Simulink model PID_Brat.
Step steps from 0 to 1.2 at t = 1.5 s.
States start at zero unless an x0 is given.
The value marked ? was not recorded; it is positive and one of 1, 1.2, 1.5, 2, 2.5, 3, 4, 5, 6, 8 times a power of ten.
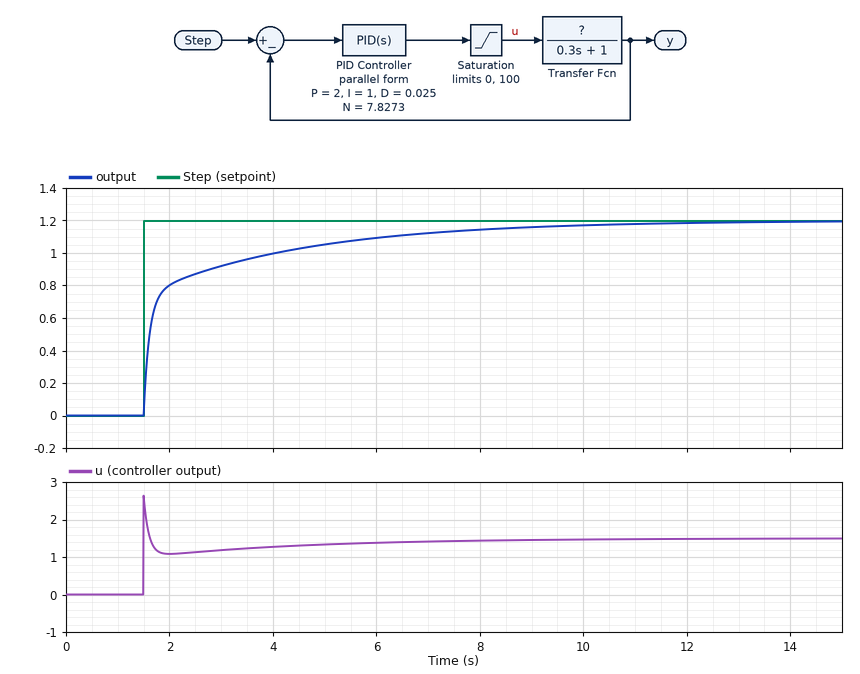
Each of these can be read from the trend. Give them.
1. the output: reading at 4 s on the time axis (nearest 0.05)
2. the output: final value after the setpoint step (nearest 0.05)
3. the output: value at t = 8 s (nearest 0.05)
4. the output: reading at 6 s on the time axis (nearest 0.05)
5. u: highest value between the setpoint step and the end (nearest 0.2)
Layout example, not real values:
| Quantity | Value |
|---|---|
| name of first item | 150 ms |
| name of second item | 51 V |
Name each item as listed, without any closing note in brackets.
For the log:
| Quantity | Value |
|---|---|
| the output: reading at 4 s on the time axis | 1.00 |
| the output: final value after the setpoint step | 1.20 |
| the output: value at t = 8 s | 1.15 |
| the output: reading at 6 s on the time axis | 1.10 |
| u: highest value between the setpoint step and the end | 2.6 |
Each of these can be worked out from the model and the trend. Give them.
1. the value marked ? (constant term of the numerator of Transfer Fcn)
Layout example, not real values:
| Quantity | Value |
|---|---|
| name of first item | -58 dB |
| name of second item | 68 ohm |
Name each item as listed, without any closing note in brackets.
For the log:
| Quantity | Value |
|---|---|
| the value marked ? | 0.8 |
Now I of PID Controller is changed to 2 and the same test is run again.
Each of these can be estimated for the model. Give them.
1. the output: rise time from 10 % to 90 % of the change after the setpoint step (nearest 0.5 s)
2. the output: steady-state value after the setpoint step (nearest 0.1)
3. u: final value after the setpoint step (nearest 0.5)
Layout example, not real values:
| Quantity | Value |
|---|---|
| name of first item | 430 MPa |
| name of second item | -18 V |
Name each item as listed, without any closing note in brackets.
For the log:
| Quantity | Value |
|---|---|
| the output: rise time from 10 % to 90 % of the change after the setpoint step | 2.0 s |
| the output: steady-state value after the setpoint step | 1.2 |
| u: final value after the setpoint step | 1.5 |
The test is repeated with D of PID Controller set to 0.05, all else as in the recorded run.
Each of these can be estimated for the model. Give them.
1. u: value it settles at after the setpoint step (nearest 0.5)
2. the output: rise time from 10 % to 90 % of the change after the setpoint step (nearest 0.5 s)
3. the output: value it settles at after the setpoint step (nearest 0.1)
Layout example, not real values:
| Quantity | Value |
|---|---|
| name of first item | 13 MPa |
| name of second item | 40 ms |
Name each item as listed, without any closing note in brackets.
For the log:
| Quantity | Value |
|---|---|
| u: value it settles at after the setpoint step | 1.5 |
| the output: rise time from 10 % to 90 % of the change after the setpoint step | 4.0 s |
| the output: value it settles at after the setpoint step | 1.2 |
